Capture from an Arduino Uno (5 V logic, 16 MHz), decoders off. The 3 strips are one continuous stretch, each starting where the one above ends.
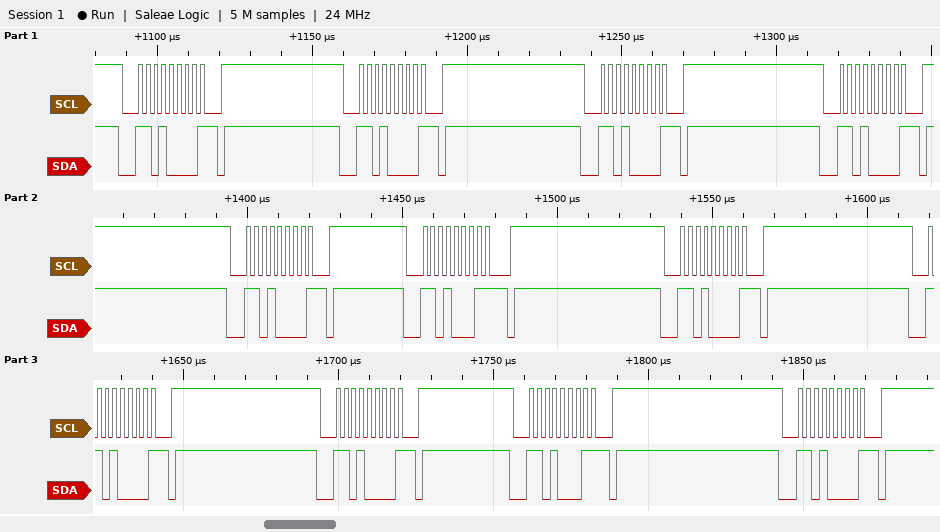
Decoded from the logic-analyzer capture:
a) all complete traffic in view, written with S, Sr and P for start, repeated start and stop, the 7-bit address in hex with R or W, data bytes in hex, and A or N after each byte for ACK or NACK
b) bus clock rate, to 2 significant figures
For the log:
S 68W N P S 68W N P S 68W N P S 68W N P S 68W N P S 68R N P S 68W N P S 68W N P S 68W N P S 68R N P S 68W N P
400 kHz
